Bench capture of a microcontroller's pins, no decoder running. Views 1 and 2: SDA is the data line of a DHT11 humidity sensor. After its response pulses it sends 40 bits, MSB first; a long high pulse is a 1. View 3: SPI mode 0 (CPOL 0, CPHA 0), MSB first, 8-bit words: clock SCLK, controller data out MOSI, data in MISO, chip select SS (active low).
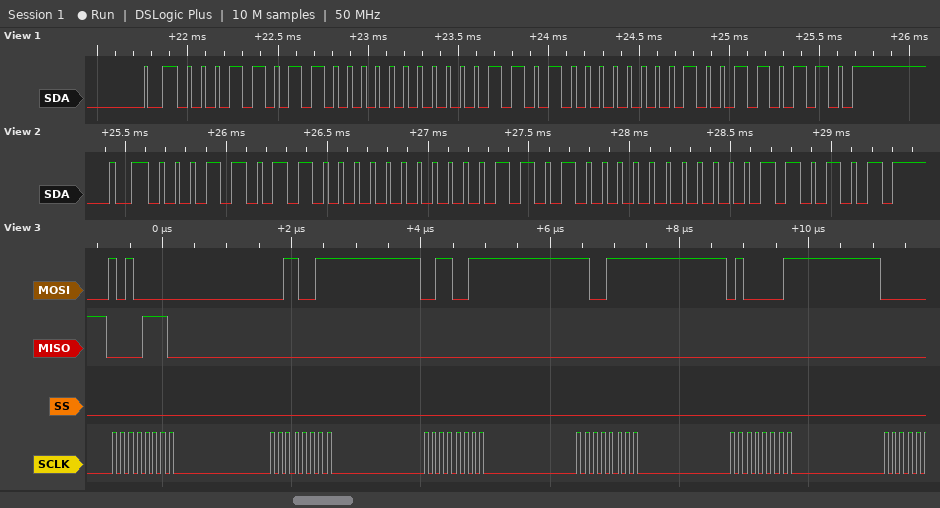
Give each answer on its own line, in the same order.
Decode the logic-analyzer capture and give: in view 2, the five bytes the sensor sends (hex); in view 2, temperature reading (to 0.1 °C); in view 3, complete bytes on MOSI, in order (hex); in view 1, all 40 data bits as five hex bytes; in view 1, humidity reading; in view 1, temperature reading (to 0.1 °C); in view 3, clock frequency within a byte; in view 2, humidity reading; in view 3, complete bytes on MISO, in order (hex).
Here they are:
1B 00 1A 00 35
26.0 °C
A0 33 33 CF 41
1B 00 1A 01 36
27 %
26.1 °C
8 MHz
27 %
0E 00 00 00 00
